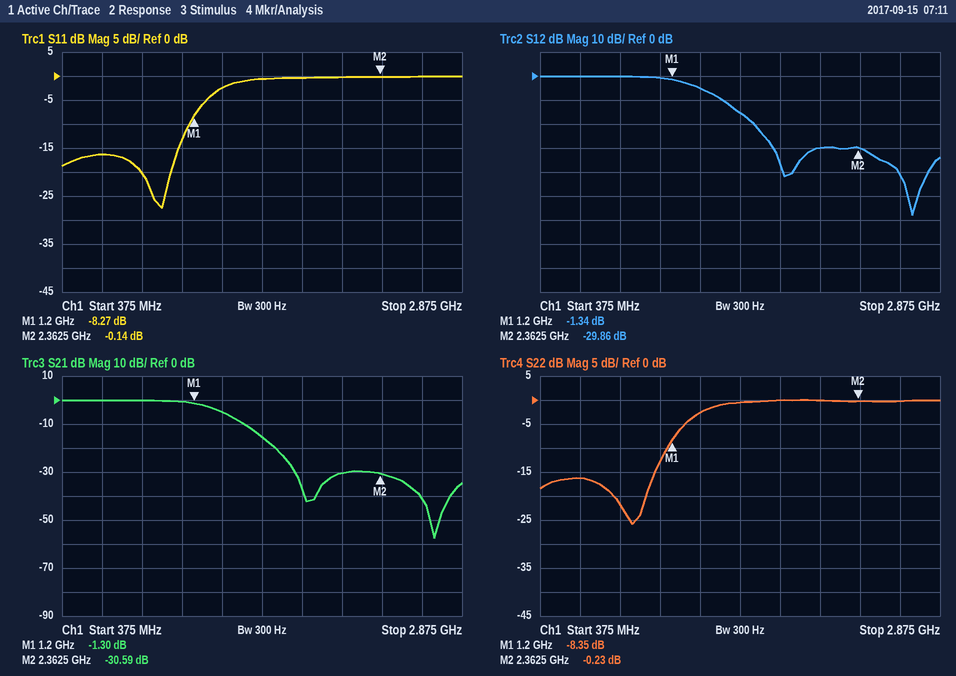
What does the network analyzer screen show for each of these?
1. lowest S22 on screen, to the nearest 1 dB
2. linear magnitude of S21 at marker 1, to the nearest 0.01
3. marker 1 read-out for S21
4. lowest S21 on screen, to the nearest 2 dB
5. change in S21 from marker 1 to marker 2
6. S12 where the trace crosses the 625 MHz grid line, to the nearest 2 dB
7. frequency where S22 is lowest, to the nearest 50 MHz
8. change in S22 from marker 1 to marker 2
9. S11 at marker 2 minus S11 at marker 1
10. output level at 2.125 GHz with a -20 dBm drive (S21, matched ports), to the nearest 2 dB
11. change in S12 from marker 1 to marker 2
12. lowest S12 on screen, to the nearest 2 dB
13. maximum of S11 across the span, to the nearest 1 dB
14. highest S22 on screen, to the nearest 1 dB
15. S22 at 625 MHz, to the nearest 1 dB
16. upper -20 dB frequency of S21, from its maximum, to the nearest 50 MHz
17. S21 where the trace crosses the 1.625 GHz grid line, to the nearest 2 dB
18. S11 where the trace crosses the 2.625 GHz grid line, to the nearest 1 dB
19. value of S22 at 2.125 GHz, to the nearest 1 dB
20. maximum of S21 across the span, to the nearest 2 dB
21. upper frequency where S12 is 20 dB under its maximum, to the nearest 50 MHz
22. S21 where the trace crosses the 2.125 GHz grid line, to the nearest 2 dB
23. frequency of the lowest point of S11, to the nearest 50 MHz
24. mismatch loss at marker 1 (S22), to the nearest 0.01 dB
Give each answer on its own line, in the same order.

-26 dB
0.86
-1.30 dB
-58 dB
-29.29 dB
0 dB
950 MHz
8.12 dB
8.13 dB
-50 dBm
-28.52 dB
-58 dB
0 dB
0 dB
-16 dB
1.70 GHz
-16 dB
0 dB
0 dB
0 dB
1.70 GHz
-30 dB
1.00 GHz
0.69 dB
